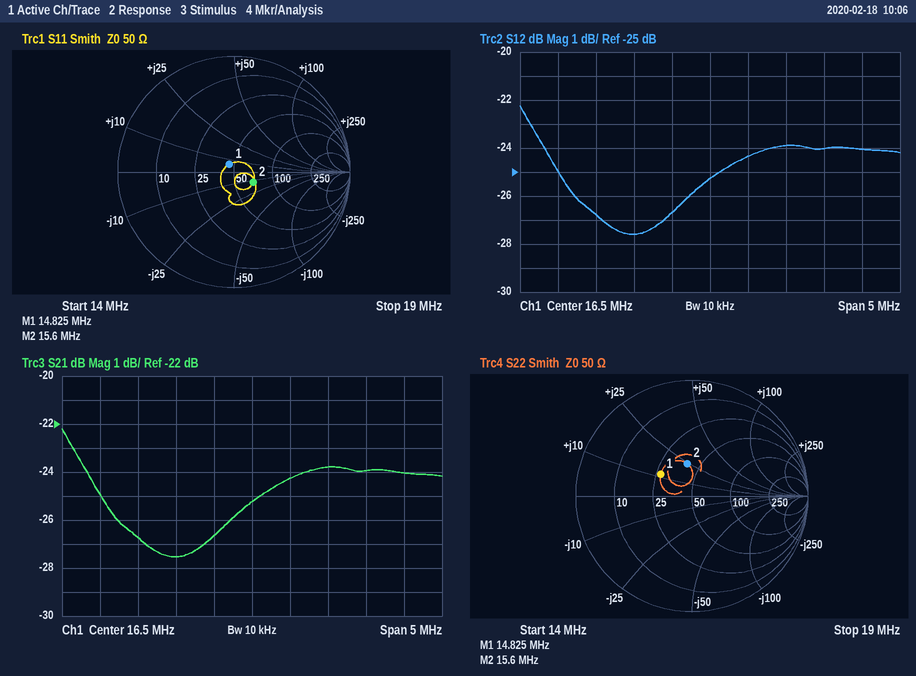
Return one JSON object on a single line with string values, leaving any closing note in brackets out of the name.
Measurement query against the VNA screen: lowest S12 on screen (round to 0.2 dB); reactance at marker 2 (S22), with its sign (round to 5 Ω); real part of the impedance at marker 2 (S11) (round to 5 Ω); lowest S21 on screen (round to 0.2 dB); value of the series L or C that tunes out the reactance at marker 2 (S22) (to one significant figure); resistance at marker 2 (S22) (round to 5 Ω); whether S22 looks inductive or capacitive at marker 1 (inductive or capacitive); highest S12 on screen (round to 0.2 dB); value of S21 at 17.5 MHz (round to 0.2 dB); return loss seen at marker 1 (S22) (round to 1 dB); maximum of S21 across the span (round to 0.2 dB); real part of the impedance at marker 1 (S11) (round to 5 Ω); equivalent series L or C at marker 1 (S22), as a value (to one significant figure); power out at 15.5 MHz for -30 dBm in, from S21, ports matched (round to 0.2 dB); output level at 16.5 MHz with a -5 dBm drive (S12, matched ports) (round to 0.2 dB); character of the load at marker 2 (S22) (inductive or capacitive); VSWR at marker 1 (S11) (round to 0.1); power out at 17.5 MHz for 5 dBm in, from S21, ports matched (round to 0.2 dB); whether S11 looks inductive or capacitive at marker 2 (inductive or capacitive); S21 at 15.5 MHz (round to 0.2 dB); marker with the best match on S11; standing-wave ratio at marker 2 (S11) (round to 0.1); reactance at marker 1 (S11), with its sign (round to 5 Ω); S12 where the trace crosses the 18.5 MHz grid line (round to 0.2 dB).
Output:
{"lowest S12 on screen": "-27.6 dB", "reactance at marker 2 (S22), with its sign": "+25 Ω", "real part of the impedance at marker 2 (S11)": "70 Ω", "lowest S21 on screen": "-27.6 dB", "value of the series L or C that tunes out the reactance at marker 2 (S22)": "400 pF", "resistance at marker 2 (S22)": "40 Ω", "whether S22 looks inductive or capacitive at marker 1": "inductive", "highest S12 on screen": "-22.2 dB", "value of S21 at 17.5 MHz": "-23.8 dB", "return loss seen at marker 1 (S22)": "10 dB", "maximum of S21 across the span": "-22.2 dB", "real part of the impedance at marker 1 (S11)": "45 Ω", "equivalent series L or C at marker 1 (S22), as a value": "100 nH", "power out at 15.5 MHz for -30 dBm in, from S21, ports matched": "-57.6 dBm", "output level at 16.5 MHz with a -5 dBm drive (S12, matched ports)": "-30.2 dBm", "character of the load at marker 2 (S22)": "inductive", "VSWR at marker 1 (S11)": "1.2", "power out at 17.5 MHz for 5 dBm in, from S21, ports matched": "-18.8 dBm", "whether S11 looks inductive or capacitive at marker 2": "capacitive", "S21 at 15.5 MHz": "-27.6 dB", "marker with the best match on S11": "marker 1", "standing-wave ratio at marker 2 (S11)": "1.5", "reactance at marker 1 (S11), with its sign": "+5 Ω", "S12 where the trace crosses the 18.5 MHz grid line": "-24.0 dB"}
